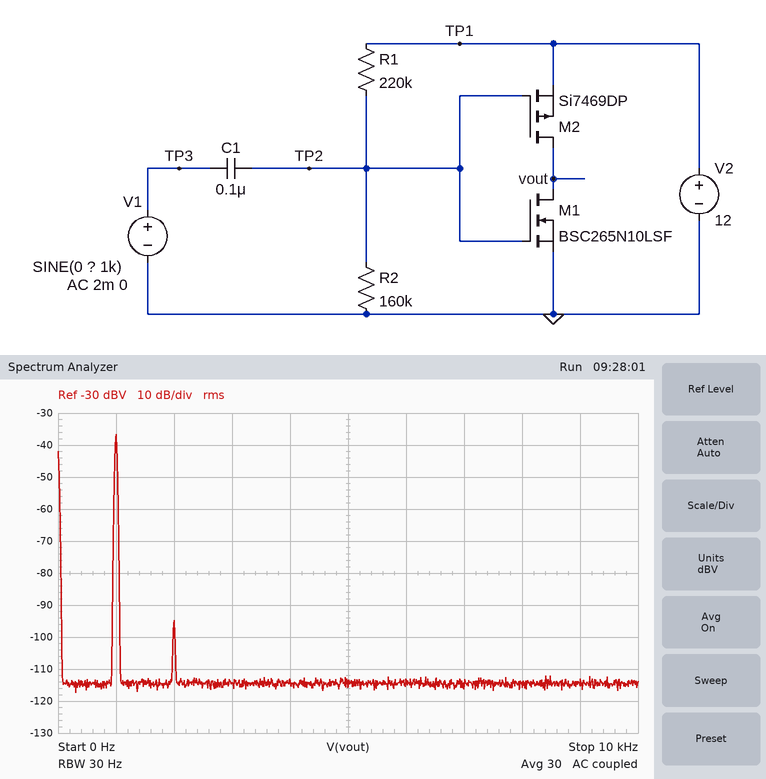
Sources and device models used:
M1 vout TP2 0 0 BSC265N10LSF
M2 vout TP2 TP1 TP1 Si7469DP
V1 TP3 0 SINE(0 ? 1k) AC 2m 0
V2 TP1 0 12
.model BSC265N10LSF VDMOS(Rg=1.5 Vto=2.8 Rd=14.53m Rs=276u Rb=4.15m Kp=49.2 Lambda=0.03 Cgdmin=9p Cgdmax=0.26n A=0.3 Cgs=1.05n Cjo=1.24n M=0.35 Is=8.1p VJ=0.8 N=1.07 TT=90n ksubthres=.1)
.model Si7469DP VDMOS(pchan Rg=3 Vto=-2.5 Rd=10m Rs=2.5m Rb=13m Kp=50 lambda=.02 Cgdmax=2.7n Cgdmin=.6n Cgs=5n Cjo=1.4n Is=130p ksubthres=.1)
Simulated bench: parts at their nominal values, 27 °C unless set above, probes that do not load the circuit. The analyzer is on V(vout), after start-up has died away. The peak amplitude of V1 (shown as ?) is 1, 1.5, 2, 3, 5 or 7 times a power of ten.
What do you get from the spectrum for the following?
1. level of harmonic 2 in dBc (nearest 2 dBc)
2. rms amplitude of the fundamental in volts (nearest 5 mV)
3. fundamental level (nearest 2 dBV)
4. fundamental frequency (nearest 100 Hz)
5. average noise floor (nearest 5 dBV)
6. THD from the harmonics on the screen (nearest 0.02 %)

-58 dBc
15 mV
-36 dBV
1.0 kHz
-115 dBV
0.12 %
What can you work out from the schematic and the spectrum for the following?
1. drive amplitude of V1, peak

10 mV
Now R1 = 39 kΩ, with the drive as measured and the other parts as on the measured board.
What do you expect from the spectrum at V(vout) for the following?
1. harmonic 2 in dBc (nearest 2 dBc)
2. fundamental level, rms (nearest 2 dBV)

-28 dBc
-92 dBV
